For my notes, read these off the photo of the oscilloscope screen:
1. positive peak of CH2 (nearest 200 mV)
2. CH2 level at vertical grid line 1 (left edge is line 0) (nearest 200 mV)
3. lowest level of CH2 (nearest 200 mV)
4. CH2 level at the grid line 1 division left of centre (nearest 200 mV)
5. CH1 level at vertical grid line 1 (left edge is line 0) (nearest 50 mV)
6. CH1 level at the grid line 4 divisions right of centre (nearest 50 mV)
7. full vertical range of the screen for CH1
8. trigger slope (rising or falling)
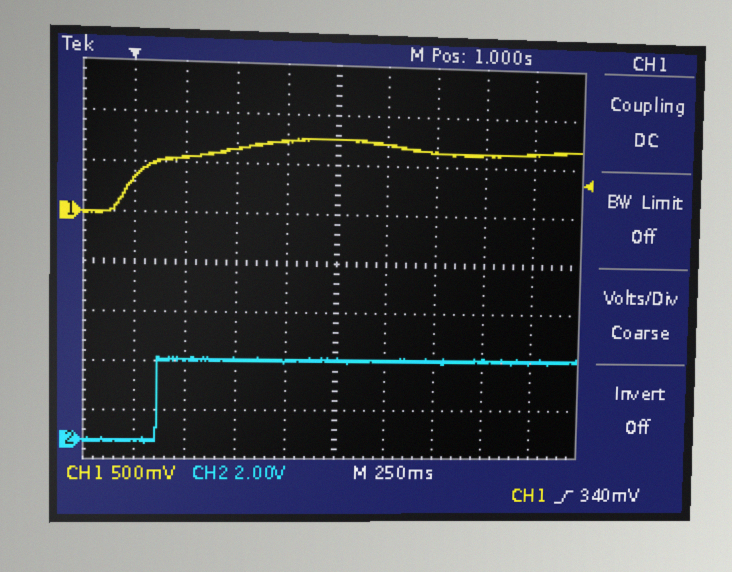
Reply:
3.4 V
0.0 V
-200 mV
3.2 V
350 mV
650 mV
4 V
rising
